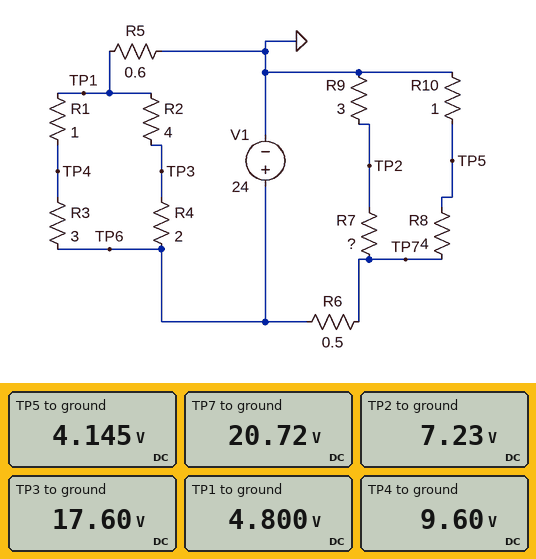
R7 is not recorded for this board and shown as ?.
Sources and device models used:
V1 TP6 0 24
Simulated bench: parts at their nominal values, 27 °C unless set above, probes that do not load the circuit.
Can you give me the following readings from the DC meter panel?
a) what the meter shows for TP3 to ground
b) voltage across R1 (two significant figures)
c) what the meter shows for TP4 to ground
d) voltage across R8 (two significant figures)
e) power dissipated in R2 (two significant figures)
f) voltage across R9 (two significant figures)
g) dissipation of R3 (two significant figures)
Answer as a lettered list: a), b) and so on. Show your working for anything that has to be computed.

a) 17.60 V
b) 9.6 V - 4.8 V = 4.8 V
c) 9.60 V
d) 20.72 V - 4.145 V = 17 V
e) (17.6 V - 4.8 V)^2 / 4 Ω = 41 W
f) 7.23 V = 7.2 V
g) (24 V - 9.6 V)^2 / 3 Ω = 69 W
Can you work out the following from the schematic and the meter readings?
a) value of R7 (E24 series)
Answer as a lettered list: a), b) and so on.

a) 5.6 Ω
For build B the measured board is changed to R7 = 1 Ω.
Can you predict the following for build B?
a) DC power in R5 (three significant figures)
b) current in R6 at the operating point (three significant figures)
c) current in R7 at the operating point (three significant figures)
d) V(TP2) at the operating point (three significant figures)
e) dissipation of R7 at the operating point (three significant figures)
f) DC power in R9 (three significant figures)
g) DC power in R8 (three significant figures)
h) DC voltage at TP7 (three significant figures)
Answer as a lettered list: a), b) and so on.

a) 38.4 W
b) 8.82 A
c) 4.90 A
d) 14.7 V
e) 24.0 W
f) 72.0 W
g) 61.4 W
h) 19.6 V
